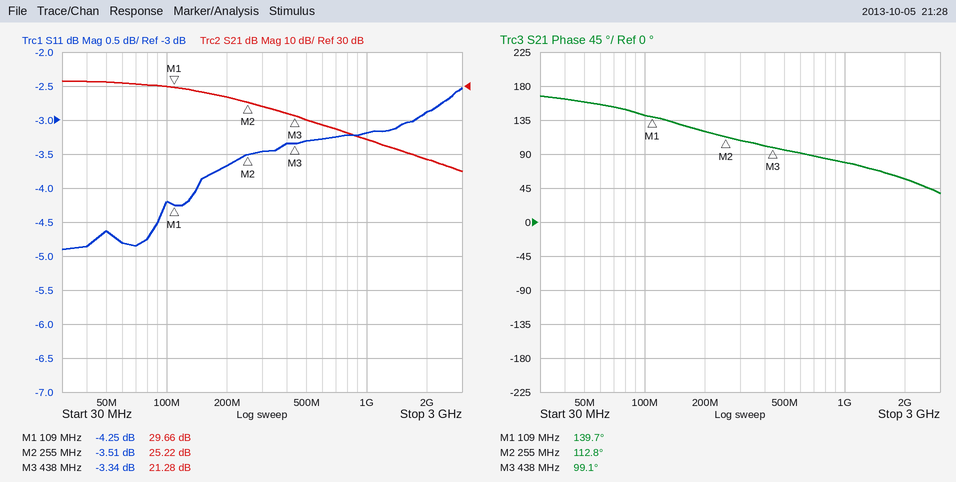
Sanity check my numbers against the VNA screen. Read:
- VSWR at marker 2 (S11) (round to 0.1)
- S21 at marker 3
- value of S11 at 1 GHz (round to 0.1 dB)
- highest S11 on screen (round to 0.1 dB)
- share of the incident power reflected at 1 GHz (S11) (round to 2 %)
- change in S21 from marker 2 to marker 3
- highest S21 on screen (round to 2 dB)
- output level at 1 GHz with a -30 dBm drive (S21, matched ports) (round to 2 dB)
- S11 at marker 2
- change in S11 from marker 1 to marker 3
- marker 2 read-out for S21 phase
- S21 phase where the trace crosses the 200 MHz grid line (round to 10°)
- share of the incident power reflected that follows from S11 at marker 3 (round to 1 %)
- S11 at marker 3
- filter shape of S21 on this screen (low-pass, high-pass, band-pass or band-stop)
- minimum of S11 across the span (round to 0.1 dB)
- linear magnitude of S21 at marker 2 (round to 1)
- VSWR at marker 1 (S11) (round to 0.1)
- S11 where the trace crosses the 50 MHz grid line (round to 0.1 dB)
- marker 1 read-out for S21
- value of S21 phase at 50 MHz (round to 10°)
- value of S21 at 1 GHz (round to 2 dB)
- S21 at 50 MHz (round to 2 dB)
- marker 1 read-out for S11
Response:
5.0
21.28 dB
-3.2 dB
-2.5 dB
48 %
-3.94 dB
32 dB
-16 dBm
-3.51 dB
0.91 dB
112.8°
120°
46 %
-3.34 dB
low-pass
-4.9 dB
18
4.2
-4.6 dB
29.66 dB
160°
14 dB
32 dB
-4.25 dB
